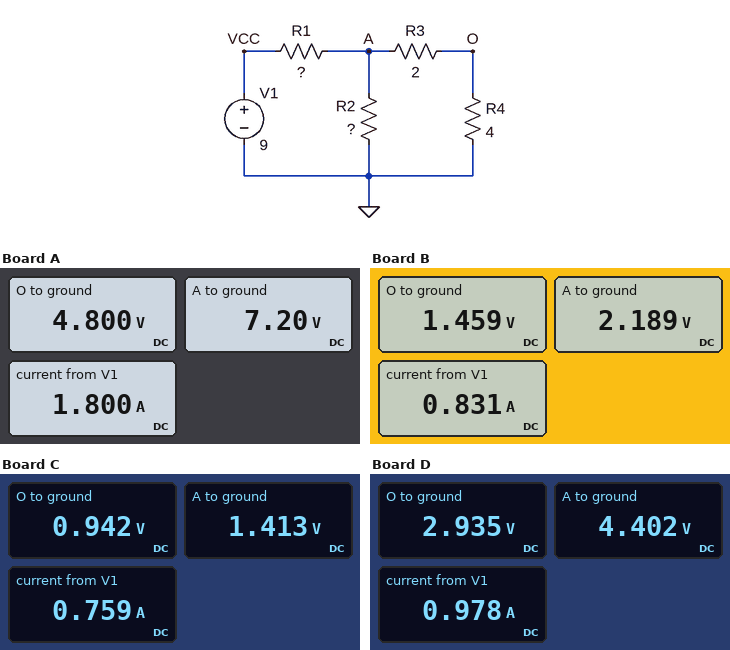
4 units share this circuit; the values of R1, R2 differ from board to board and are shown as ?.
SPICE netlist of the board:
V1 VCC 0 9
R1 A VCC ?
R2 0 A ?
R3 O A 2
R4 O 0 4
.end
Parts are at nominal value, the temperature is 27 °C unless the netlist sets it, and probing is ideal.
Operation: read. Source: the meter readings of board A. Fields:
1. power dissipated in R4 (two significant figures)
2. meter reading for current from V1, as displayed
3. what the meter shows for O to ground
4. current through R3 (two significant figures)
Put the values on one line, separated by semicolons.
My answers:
5.8 W; 1.800 A; 4.800 V; 1.2 A
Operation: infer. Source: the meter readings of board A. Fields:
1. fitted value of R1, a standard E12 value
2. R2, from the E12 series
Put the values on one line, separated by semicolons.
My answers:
1 Ω; 12 Ω
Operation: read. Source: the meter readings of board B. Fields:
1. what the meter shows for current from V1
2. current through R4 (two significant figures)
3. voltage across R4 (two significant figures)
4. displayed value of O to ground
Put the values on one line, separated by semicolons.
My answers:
0.831 A; 360 mA; 1.5 V; 1.459 V
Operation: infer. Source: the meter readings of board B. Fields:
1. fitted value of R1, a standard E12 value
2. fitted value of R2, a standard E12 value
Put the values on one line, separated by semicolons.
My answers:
8.2 Ω; 4.7 Ω
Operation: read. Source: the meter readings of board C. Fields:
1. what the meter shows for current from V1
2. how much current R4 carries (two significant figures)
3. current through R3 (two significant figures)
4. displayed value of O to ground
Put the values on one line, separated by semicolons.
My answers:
0.759 A; 240 mA; 240 mA; 0.942 V
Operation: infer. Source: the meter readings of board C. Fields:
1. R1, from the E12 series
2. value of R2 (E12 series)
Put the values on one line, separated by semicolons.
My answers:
10 Ω; 2.7 Ω
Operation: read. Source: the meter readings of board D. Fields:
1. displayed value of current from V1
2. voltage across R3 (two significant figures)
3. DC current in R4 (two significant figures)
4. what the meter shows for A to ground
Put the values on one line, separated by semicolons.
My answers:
0.978 A; 1.5 V; 730 mA; 4.402 V
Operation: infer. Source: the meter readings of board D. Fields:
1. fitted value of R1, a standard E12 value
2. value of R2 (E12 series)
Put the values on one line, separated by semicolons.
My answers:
4.7 Ω; 18 Ω
